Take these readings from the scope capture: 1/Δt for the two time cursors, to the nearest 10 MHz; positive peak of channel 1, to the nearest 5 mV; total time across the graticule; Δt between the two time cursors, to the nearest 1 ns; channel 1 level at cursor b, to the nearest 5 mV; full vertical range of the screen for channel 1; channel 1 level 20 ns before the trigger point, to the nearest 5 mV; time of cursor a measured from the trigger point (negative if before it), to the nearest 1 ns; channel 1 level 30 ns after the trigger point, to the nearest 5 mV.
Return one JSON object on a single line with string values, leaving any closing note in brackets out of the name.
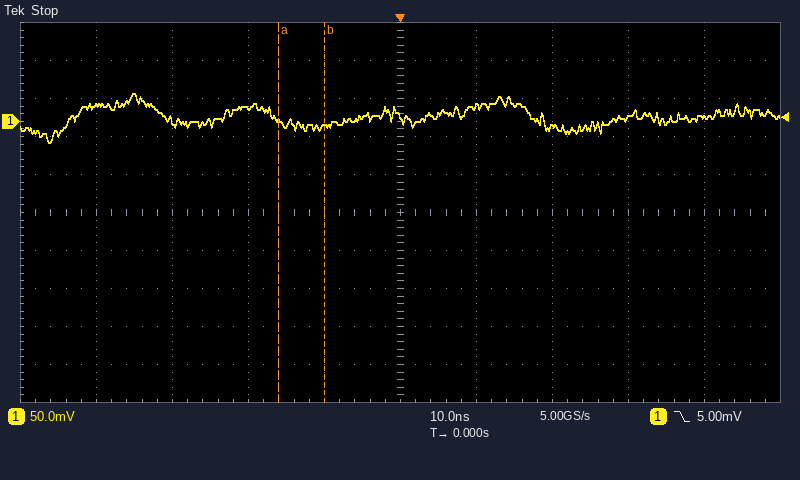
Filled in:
{"1/Δt for the two time cursors, to the nearest 10 MHz": "170 MHz", "positive peak of channel 1, to the nearest 5 mV": "35 mV", "total time across the graticule": "100 ns", "Δt between the two time cursors, to the nearest 1 ns": "6 ns", "channel 1 level at cursor b, to the nearest 5 mV": "-5 mV", "full vertical range of the screen for channel 1": "500 mV", "channel 1 level 20 ns before the trigger point, to the nearest 5 mV": "20 mV", "time of cursor a measured from the trigger point (negative if before it), to the nearest 1 ns": "-16 ns", "channel 1 level 30 ns after the trigger point, to the nearest 5 mV": "5 mV"}
